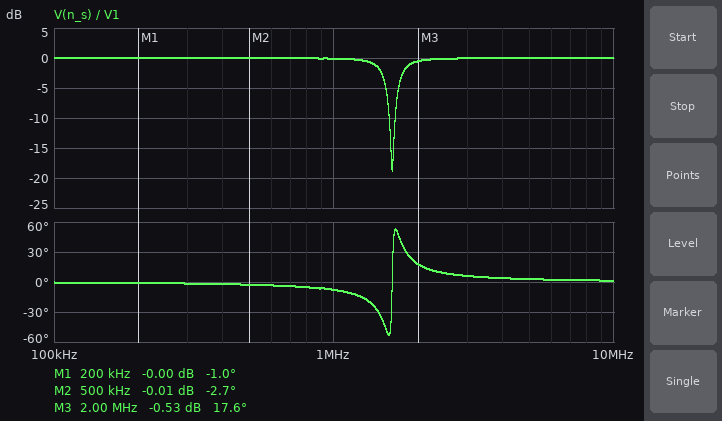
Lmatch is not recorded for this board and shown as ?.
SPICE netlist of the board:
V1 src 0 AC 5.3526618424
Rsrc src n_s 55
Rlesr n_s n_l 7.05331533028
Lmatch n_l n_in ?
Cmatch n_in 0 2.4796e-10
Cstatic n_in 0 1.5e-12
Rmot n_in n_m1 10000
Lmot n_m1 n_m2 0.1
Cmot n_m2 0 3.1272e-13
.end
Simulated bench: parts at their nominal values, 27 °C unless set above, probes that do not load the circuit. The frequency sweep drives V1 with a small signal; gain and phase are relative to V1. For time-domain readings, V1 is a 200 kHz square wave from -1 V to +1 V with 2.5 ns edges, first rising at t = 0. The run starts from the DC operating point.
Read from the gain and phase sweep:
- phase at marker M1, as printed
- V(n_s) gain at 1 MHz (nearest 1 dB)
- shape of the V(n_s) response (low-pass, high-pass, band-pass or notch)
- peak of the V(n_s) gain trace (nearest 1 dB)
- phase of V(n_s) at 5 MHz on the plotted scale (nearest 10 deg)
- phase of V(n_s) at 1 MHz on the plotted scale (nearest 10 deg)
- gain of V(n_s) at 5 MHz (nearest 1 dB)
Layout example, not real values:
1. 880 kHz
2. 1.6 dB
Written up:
1. -1.0 deg
2. 0 dB
3. notch
4. 0 dB
5. 0 deg
6. -10 deg
7. 0 dB
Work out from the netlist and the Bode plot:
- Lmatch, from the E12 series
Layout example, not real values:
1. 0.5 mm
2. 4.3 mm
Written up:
1. 39 µH
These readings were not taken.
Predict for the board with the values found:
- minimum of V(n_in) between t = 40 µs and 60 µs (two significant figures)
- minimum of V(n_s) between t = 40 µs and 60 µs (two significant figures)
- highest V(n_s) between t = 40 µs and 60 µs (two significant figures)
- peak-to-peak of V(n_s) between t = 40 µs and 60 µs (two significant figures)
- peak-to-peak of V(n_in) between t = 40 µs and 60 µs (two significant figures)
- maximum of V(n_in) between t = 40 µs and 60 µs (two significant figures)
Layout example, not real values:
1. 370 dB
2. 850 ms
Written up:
1. -2.4 V
2. -1.2 V
3. 1.2 V
4. 2.3 V
5. 4.7 V
6. 2.4 V
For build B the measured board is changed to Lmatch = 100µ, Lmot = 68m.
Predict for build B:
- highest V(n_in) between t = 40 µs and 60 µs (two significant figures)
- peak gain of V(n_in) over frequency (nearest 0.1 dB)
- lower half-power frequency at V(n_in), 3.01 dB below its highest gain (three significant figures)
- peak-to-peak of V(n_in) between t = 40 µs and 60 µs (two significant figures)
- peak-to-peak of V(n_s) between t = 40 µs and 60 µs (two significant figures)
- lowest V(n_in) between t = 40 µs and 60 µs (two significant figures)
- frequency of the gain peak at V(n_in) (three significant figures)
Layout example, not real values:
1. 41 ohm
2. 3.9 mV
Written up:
1. 4.2 V
2. 20.1 dB
3. 951 kHz
4. 8.3 V
5. 2.5 V
6. -4.2 V
7. 1.00 MHz
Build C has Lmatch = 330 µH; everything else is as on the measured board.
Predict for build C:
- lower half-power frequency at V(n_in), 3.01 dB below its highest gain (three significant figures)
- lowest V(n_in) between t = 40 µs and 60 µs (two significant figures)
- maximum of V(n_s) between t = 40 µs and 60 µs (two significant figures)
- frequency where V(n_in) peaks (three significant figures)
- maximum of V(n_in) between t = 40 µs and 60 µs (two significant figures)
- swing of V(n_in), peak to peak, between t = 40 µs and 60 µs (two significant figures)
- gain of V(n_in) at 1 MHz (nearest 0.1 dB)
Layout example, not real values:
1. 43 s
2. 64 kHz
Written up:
1. 539 kHz
2. -3.7 V
3. 1.1 V
4. 554 kHz
5. 3.7 V
6. 7.4 V
7. -7.0 dB
